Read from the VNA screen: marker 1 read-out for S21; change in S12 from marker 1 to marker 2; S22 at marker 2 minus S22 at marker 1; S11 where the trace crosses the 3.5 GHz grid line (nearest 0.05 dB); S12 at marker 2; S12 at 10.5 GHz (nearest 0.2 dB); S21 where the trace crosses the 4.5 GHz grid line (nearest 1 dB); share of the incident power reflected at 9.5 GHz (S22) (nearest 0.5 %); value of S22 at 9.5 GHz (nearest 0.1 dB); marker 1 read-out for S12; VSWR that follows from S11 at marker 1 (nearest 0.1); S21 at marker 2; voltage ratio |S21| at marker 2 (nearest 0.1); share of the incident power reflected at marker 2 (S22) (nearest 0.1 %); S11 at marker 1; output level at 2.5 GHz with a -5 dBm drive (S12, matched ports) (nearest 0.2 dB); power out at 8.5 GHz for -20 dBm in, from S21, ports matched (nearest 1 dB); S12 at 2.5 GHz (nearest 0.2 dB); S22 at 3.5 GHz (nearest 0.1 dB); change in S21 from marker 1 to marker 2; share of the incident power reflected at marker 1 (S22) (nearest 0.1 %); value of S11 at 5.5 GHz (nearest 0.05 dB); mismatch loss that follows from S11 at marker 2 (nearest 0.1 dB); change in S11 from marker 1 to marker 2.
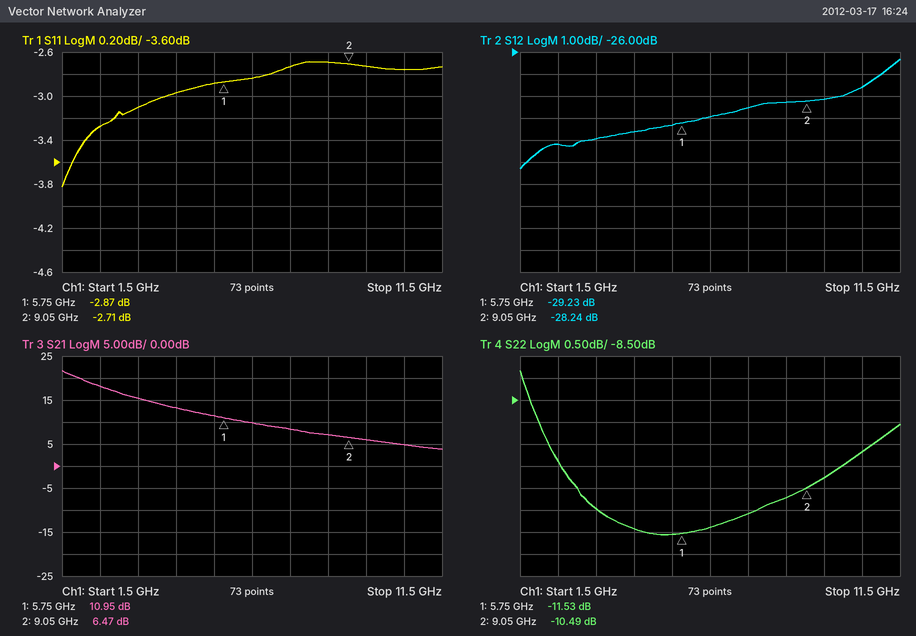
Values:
10.95 dB
0.99 dB
1.04 dB
-3.10 dB
-28.24 dB
-27.6 dB
13 dB
9.5 %
-10.3 dB
-29.23 dB
6.1
6.47 dB
2.1
8.9 %
-2.87 dB
-35.2 dBm
-13 dBm
-30.2 dB
-11.0 dB
-4.48 dB
7.0 %
-2.90 dB
3.3 dB
0.16 dB
